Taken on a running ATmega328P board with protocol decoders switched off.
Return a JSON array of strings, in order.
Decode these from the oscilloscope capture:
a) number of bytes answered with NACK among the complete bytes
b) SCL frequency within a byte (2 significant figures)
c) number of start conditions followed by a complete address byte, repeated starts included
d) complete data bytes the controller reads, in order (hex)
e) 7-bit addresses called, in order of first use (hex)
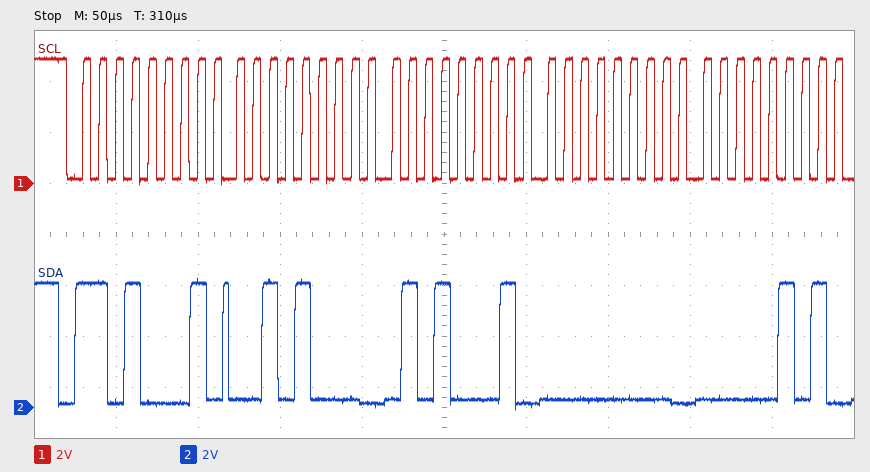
["0", "100 kHz", "1", "28 51 00 05", "0x68"]
